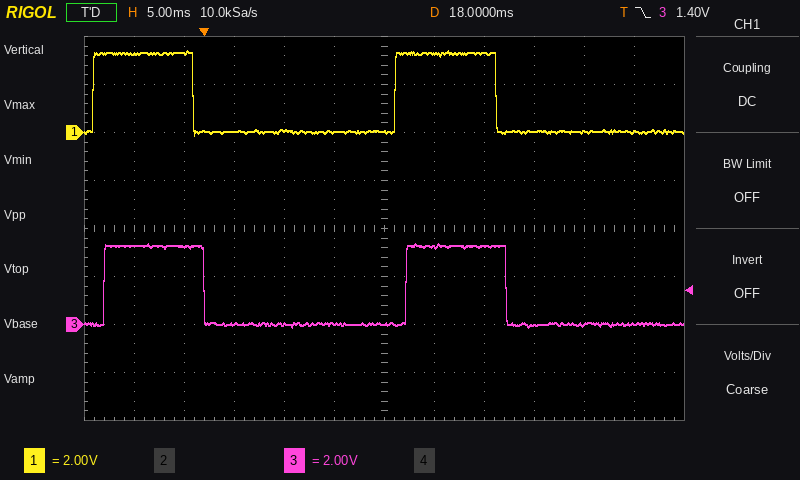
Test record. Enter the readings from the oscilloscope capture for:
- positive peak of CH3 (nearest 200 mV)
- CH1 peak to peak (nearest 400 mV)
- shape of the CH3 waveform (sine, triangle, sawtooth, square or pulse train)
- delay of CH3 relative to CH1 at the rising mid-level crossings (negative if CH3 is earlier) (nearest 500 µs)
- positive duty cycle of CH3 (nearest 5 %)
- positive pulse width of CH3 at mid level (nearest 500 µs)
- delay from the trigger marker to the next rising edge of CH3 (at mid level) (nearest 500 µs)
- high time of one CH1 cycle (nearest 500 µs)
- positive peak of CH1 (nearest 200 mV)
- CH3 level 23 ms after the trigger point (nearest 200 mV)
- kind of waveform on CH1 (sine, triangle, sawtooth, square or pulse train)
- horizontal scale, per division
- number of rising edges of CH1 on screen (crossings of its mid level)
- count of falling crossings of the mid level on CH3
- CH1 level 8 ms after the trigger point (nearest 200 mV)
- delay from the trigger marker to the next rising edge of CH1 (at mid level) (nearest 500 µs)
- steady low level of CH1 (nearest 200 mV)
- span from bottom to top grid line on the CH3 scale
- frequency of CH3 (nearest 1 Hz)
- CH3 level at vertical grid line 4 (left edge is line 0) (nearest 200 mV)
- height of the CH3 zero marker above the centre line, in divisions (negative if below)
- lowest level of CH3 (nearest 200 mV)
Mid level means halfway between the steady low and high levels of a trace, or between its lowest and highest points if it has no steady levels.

3.4 V
3.6 V
pulse train
+1.0 ms
35 %
10.0 ms
20.0 ms
10.0 ms
3.4 V
3.2 V
pulse train
5 ms
2
2
0.0 V
19.0 ms
0.0 V
16 V
33 Hz
0.0 V
-2.0 div
-200 mV
